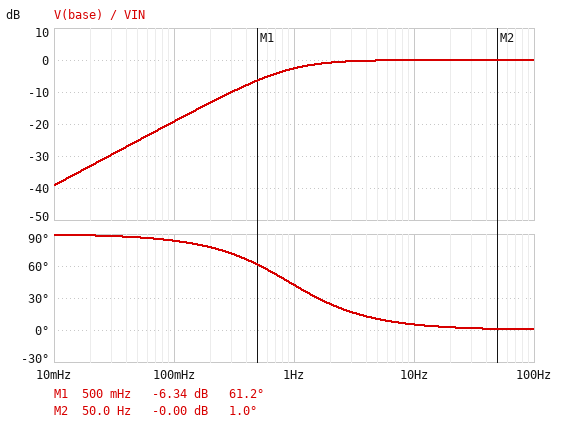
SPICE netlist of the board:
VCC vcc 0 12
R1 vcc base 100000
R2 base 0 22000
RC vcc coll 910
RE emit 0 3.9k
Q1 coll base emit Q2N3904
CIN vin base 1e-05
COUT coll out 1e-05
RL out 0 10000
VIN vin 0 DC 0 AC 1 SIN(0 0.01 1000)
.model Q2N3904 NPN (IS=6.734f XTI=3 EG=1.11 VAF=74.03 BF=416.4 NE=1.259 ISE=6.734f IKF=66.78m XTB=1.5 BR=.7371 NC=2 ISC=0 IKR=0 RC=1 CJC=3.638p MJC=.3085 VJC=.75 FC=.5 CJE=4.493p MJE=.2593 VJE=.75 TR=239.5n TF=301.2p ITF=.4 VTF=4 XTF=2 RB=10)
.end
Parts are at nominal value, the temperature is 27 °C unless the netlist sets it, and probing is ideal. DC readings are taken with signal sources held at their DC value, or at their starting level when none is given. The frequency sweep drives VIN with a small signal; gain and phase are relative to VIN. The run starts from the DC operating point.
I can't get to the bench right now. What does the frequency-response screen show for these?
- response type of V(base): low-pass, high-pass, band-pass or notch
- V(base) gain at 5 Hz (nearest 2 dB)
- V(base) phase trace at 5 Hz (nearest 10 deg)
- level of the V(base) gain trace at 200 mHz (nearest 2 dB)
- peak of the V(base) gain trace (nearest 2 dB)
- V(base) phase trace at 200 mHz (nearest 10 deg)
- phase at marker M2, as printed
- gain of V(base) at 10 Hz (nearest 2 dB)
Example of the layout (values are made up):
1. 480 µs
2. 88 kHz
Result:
1. high-pass
2. 0 dB
3. 10 deg
4. -14 dB
5. 0 dB
6. 80 deg
7. 1.0 deg
8. 0 dB
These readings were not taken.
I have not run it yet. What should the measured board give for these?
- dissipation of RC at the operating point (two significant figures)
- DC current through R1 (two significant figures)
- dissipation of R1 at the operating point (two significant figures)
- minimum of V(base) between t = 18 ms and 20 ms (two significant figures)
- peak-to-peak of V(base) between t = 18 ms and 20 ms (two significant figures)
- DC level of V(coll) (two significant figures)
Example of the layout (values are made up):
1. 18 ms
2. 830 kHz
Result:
1. 130 µW
2. 99 µA
3. 980 µW
4. 2.1 V
5. 20 mV
6. 12 V
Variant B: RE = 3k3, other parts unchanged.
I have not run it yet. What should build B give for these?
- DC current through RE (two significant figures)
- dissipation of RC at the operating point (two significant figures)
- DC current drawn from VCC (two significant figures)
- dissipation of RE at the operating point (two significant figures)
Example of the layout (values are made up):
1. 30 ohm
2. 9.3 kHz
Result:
1. 440 µA
2. 180 µW
3. 540 µA
4. 650 µW
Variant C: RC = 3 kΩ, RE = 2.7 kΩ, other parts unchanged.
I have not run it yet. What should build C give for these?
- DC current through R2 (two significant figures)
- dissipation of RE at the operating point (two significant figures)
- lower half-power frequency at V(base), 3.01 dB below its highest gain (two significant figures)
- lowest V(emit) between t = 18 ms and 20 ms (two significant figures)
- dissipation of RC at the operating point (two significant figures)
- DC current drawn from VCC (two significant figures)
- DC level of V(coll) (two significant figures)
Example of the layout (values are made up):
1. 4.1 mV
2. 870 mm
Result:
1. 95 µA
2. 770 µW
3. 920 mHz
4. 1.4 V
5. 850 µW
6. 630 µA
7. 10 V
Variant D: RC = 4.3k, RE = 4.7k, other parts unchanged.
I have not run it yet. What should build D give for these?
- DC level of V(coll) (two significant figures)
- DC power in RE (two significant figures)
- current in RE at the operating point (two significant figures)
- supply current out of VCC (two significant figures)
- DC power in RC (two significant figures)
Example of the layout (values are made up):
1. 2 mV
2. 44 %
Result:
1. 11 V
2. 470 µW
3. 320 µA
4. 410 µA
5. 420 µW
